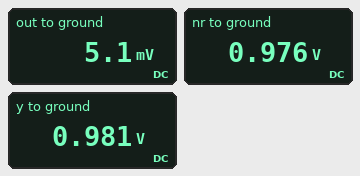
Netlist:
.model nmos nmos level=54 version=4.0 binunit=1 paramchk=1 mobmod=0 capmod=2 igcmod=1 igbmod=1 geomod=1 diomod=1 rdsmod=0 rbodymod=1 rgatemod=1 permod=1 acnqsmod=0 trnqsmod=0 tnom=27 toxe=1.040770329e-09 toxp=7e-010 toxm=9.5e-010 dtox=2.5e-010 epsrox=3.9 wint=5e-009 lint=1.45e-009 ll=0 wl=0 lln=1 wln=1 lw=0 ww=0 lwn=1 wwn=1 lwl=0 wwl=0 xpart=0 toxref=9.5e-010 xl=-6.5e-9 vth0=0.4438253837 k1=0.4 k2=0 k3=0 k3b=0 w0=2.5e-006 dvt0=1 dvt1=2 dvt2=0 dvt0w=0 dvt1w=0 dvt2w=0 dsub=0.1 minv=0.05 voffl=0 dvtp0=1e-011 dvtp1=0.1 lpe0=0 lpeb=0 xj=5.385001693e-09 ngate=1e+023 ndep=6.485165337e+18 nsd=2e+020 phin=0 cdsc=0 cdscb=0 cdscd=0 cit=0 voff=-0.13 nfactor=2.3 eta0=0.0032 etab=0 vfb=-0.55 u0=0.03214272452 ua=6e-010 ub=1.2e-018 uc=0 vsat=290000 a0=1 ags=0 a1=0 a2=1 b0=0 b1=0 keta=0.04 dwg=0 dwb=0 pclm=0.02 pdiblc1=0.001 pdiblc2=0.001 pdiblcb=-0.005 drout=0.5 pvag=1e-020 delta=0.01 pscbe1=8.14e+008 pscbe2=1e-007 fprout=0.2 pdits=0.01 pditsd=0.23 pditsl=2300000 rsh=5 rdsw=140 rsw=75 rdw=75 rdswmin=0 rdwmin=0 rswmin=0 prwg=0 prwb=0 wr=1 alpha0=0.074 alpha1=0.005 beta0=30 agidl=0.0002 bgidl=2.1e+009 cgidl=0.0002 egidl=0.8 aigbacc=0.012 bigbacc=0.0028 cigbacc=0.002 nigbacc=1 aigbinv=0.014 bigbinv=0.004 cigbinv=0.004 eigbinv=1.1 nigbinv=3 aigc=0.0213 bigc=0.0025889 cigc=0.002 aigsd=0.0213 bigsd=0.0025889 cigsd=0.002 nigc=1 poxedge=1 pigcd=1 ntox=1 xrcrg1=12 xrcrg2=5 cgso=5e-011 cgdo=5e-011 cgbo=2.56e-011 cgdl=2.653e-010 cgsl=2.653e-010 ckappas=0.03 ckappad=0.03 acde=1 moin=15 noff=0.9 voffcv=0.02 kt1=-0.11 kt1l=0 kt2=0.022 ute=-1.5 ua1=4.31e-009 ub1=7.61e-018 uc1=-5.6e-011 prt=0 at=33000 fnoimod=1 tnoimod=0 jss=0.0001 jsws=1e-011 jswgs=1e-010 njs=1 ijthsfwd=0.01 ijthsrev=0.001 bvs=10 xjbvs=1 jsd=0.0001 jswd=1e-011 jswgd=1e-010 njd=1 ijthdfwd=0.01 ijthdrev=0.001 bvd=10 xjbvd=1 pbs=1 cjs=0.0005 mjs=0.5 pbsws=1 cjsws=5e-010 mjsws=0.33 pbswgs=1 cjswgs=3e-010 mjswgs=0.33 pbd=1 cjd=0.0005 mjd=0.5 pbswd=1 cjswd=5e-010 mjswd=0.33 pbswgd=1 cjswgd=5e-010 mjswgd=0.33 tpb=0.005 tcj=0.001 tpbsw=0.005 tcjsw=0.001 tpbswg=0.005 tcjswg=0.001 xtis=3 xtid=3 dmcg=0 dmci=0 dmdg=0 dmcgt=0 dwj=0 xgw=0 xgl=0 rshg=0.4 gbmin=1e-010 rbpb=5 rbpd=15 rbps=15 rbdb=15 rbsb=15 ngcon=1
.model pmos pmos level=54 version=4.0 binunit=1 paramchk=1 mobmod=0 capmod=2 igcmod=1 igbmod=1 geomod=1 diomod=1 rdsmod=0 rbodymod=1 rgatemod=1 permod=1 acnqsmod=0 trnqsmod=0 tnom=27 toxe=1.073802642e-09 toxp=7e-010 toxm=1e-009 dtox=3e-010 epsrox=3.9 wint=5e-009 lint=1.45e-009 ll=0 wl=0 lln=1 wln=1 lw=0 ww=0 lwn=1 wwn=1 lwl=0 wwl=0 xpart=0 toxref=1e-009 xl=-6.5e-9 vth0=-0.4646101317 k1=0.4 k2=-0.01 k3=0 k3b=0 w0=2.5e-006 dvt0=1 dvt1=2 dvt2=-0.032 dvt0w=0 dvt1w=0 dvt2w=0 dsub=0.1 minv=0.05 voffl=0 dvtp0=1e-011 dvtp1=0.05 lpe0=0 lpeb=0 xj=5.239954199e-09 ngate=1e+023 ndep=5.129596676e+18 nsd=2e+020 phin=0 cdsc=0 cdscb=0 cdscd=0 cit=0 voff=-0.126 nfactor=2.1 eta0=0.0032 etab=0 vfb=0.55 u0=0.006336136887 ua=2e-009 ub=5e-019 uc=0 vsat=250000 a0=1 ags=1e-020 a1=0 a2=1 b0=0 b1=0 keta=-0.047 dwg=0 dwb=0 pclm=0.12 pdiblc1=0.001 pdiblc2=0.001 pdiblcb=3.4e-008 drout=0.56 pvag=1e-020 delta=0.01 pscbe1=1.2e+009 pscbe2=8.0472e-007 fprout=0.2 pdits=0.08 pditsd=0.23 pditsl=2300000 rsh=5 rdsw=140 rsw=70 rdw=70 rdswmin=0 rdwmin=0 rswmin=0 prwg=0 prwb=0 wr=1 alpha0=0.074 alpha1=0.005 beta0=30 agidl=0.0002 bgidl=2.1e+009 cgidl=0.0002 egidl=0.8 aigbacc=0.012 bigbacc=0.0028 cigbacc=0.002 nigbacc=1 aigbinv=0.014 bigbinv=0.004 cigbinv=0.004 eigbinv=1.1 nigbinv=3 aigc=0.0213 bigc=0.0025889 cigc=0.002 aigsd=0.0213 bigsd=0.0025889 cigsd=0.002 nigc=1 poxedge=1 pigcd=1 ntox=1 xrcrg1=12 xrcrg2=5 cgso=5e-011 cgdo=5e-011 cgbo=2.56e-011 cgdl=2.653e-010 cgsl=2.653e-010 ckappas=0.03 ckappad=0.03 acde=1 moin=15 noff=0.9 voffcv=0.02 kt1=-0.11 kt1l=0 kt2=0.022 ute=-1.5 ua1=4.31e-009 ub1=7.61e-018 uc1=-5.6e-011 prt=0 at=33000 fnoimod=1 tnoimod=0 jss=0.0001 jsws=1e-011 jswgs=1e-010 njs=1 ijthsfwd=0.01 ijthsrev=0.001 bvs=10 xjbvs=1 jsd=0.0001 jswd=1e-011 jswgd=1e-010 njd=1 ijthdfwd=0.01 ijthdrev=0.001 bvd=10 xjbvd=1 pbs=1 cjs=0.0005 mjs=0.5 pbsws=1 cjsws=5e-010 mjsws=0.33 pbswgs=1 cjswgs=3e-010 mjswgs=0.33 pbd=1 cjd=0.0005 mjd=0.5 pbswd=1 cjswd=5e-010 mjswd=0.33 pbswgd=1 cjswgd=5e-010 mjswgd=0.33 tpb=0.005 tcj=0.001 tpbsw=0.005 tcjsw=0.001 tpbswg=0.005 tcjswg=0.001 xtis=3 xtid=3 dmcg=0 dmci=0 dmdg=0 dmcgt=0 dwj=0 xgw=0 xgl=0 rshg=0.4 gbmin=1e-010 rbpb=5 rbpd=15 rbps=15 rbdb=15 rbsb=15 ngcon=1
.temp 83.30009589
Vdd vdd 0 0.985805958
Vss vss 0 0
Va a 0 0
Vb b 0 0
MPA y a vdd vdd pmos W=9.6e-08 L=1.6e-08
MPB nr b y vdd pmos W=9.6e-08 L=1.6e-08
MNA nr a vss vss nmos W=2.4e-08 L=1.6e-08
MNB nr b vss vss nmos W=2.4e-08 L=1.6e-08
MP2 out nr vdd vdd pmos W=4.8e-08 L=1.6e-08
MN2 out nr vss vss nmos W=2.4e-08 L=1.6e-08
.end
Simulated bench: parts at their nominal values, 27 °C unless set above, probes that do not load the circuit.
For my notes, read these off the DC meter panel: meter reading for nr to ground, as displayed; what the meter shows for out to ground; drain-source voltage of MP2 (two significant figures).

0.976 V
5.1 mV
-980 mV
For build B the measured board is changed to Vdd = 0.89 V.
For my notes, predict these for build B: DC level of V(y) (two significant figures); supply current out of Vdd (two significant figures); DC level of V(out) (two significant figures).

890 mV
480 nA
1.9 mV
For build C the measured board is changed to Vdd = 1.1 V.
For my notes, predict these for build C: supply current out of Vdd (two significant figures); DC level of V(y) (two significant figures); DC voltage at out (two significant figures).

3.0 µA
1.1 V
17 mV
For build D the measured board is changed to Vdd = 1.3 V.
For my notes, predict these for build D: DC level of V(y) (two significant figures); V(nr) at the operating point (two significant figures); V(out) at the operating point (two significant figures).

1.3 V
1.2 V
96 mV
